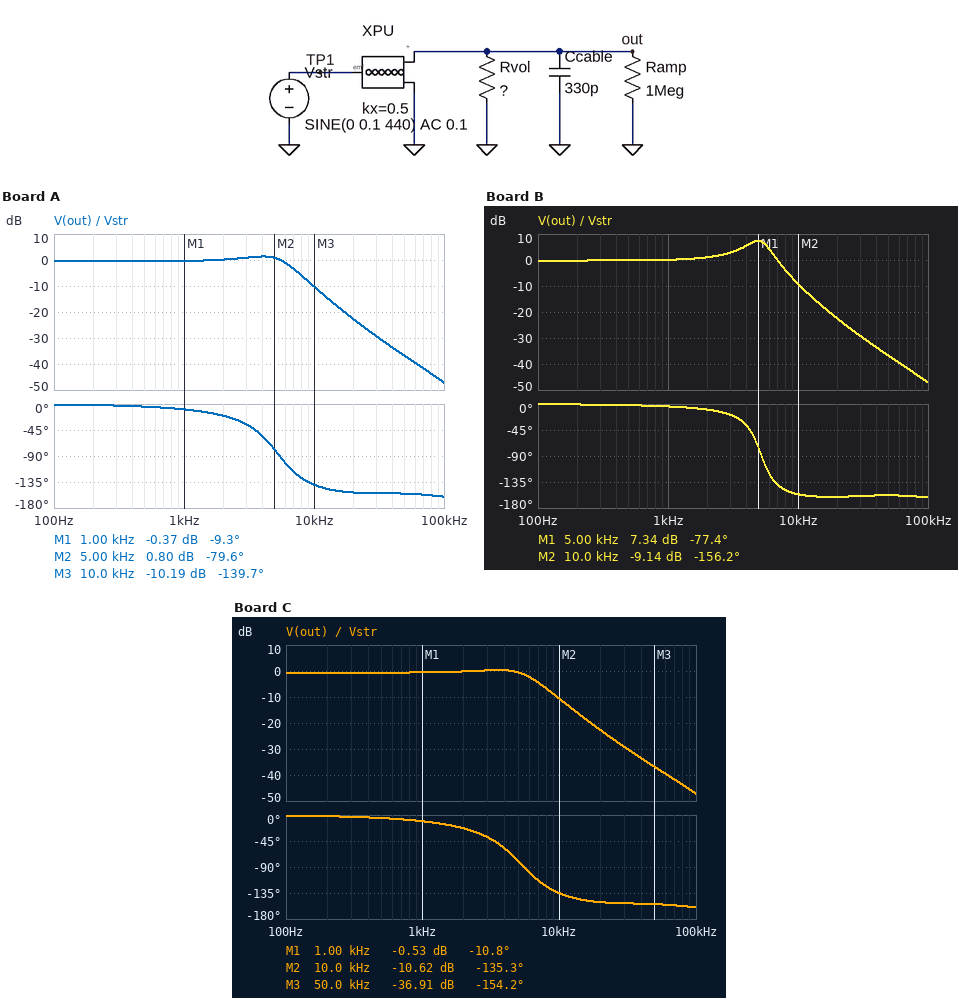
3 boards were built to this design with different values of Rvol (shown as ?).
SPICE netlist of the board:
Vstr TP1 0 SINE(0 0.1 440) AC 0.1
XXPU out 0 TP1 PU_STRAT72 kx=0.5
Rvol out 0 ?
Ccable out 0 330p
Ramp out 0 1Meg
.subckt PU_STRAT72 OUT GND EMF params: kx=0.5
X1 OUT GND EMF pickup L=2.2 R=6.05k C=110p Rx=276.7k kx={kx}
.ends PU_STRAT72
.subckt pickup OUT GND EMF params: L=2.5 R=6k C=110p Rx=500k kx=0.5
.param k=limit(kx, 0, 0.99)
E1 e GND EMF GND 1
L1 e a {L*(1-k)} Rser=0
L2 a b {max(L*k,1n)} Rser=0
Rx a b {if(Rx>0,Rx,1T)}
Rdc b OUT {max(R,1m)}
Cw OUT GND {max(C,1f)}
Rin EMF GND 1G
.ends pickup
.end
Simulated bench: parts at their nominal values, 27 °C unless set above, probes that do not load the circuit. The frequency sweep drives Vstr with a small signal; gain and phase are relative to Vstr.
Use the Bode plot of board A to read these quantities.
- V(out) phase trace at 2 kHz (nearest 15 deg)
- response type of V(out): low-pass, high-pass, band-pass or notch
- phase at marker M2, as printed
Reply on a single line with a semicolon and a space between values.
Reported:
-15 deg; low-pass; -79.6 deg
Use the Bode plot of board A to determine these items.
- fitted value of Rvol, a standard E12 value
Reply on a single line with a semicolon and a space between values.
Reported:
100 kΩ
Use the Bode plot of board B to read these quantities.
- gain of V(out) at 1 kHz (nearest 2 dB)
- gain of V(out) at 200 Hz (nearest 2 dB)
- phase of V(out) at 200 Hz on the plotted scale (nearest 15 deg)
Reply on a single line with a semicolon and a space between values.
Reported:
0 dB; 0 dB; 0 deg
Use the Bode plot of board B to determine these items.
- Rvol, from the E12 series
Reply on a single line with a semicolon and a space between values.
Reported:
330 kΩ
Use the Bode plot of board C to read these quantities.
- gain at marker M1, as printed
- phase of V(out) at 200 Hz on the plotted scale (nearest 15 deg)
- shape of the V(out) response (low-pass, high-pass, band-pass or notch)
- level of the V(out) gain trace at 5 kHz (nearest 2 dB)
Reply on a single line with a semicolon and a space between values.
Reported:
-0.53 dB; 0 deg; low-pass; 0 dB
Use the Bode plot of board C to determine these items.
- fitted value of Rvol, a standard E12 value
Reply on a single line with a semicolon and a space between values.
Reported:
82 kΩ
